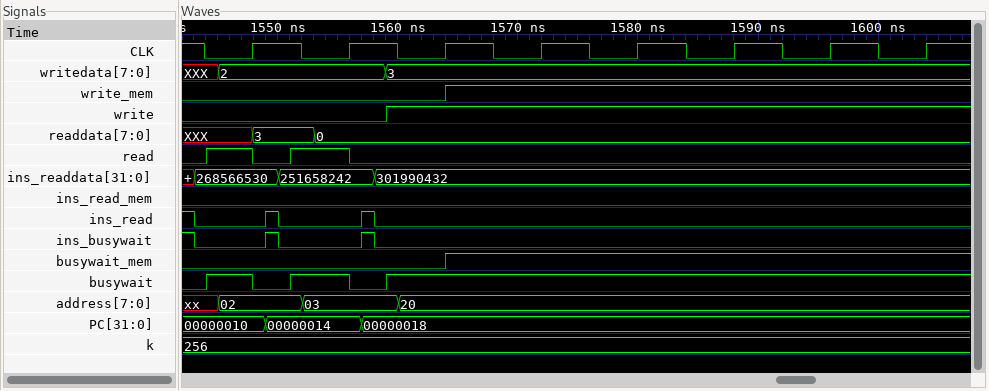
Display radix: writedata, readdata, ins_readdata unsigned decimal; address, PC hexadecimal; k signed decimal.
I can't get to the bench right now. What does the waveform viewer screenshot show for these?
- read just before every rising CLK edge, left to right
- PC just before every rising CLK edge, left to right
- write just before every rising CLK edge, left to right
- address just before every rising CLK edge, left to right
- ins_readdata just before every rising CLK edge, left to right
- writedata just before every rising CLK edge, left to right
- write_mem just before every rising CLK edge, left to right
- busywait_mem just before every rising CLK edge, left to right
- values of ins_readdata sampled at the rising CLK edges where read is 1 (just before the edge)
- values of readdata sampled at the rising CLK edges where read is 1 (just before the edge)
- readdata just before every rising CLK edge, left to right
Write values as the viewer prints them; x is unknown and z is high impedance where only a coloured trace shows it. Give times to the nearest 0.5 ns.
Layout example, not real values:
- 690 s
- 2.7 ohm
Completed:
- 1 1 0 0 0 0 0 0
- 00000010, 00000014, 00000018, 00000018, 00000018, 00000018, 00000018, 00000018
- 0 0 1 1 1 1 1 1
- 02, 03, 20, 20, 20, 20, 20, 20
- 268566530, 251658242, 301990432, 301990432, 301990432, 301990432, 301990432, 301990432
- 2, 2, 3, 3, 3, 3, 3, 3
- 0 0 0 1 1 1 1 1
- 0 0 0 1 1 1 1 1
- 268566530, 251658242
- XXX, 0
- XXX, 0, 0, 0, 0, 0, 0, 0
